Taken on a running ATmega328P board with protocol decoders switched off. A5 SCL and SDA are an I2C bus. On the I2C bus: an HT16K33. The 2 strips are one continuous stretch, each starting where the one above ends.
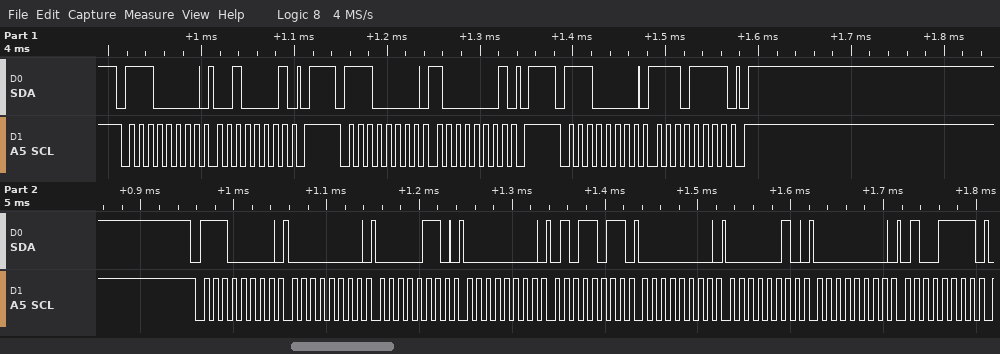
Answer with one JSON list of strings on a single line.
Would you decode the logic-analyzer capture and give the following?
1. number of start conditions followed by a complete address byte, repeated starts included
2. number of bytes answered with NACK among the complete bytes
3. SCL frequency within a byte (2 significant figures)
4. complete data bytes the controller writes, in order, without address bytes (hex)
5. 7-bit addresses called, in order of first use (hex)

["4", "0", "100 kHz", "21 81 EF 00 06 00 5B 00 02 00 4F", "0x70"]
